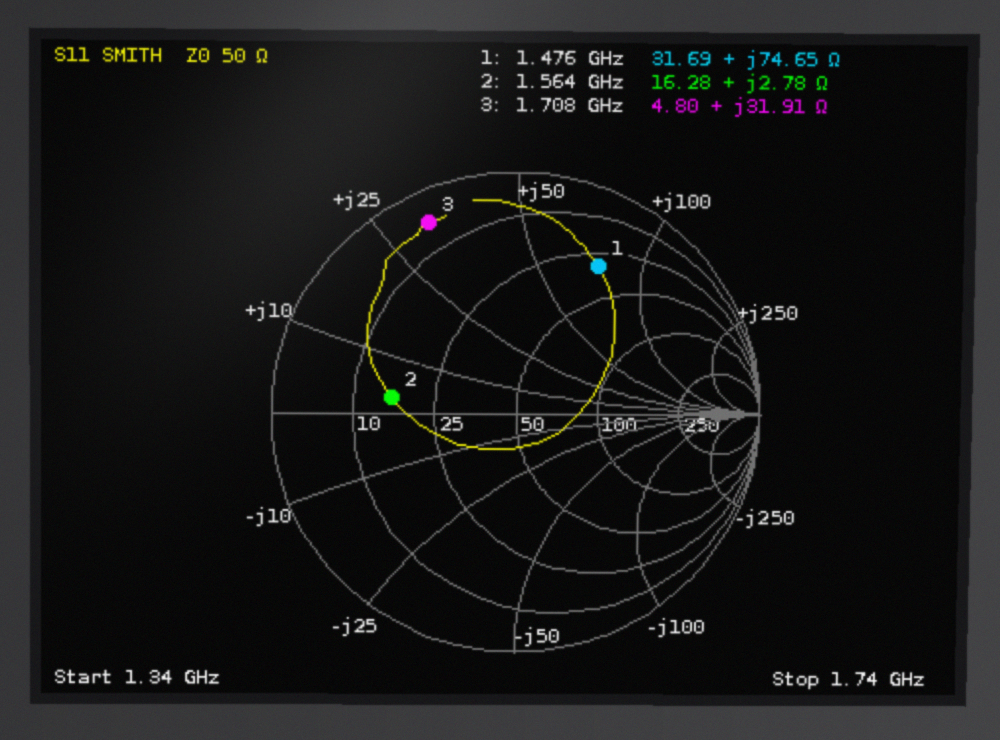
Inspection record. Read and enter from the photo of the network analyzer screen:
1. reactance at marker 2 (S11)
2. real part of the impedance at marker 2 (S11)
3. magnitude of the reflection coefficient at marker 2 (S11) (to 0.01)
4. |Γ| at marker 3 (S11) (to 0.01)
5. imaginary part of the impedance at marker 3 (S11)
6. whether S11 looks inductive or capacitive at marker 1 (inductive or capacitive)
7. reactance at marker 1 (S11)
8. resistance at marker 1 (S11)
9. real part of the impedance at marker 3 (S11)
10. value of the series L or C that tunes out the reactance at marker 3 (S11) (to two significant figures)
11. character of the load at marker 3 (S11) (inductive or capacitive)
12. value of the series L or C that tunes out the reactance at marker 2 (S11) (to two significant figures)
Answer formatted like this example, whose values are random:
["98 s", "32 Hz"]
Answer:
["+2.78 Ω", "16.28 Ω", "0.51", "0.87", "+31.91 Ω", "inductive", "+74.65 Ω", "31.69 Ω", "4.80 Ω", "2.9 pF", "inductive", "37 pF"]
